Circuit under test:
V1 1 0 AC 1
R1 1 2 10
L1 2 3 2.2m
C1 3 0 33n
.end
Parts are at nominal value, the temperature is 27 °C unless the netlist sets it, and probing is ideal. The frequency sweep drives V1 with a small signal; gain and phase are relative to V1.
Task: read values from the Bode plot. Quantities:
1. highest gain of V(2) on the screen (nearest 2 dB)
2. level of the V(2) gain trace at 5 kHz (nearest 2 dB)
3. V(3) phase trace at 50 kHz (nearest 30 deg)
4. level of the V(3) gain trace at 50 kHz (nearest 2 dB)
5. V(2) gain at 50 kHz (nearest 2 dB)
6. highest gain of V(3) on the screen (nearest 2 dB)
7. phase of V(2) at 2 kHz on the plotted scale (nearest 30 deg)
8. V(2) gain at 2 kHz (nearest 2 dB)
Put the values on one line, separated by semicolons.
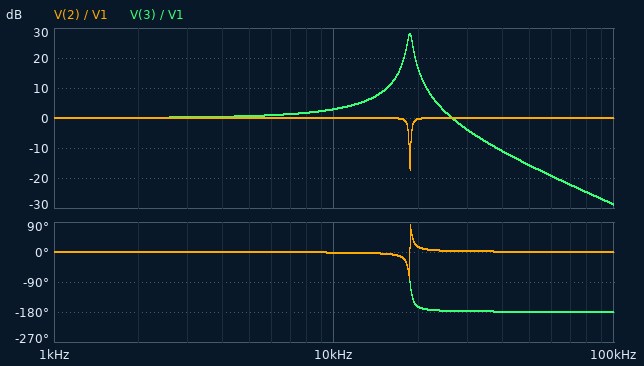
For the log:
0 dB; 0 dB; -180 deg; -16 dB; 0 dB; 28 dB; 0 deg; 0 dB
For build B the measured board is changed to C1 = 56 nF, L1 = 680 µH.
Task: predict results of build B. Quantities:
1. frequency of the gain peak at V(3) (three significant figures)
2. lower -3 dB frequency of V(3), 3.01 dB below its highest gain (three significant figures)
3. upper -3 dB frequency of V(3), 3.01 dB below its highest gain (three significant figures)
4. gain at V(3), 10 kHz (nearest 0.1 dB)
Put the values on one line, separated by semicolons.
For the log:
25.7 kHz; 24.5 kHz; 26.9 kHz; 1.4 dB
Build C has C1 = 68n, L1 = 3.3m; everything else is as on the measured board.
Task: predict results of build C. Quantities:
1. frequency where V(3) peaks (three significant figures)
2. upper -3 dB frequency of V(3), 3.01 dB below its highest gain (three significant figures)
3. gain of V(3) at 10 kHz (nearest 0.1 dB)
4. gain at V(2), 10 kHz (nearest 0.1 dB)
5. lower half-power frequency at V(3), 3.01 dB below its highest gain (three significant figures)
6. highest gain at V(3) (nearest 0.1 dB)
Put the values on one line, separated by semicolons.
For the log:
10.6 kHz; 10.9 kHz; 18.3 dB; -0.6 dB; 10.4 kHz; 26.9 dB
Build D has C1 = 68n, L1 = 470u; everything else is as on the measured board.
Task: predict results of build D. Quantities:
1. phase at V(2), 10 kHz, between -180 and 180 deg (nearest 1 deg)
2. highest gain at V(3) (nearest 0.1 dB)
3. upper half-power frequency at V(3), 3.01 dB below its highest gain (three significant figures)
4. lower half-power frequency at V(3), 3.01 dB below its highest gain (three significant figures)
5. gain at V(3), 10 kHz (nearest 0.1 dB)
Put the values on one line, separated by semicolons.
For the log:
-3 deg; 18.4 dB; 29.7 kHz; 26.3 kHz; 1.2 dB
